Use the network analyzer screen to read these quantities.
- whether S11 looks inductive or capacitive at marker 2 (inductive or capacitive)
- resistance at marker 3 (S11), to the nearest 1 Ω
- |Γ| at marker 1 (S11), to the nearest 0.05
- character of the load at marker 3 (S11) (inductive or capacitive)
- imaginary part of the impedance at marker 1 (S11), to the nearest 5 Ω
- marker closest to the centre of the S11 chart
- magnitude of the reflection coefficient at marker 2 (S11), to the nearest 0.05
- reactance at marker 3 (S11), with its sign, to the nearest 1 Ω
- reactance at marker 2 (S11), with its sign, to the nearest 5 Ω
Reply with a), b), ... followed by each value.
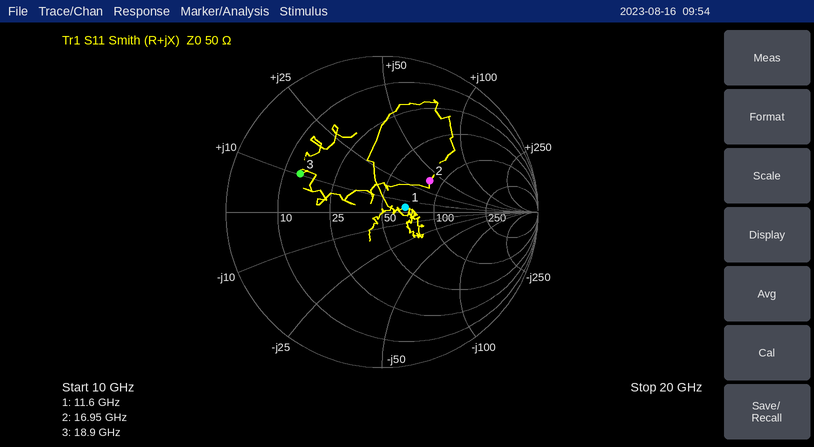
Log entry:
a) inductive
b) 14 Ω
c) 0.15
d) inductive
e) +5 Ω
f) marker 1
g) 0.35
h) +10 Ω
i) +40 Ω
